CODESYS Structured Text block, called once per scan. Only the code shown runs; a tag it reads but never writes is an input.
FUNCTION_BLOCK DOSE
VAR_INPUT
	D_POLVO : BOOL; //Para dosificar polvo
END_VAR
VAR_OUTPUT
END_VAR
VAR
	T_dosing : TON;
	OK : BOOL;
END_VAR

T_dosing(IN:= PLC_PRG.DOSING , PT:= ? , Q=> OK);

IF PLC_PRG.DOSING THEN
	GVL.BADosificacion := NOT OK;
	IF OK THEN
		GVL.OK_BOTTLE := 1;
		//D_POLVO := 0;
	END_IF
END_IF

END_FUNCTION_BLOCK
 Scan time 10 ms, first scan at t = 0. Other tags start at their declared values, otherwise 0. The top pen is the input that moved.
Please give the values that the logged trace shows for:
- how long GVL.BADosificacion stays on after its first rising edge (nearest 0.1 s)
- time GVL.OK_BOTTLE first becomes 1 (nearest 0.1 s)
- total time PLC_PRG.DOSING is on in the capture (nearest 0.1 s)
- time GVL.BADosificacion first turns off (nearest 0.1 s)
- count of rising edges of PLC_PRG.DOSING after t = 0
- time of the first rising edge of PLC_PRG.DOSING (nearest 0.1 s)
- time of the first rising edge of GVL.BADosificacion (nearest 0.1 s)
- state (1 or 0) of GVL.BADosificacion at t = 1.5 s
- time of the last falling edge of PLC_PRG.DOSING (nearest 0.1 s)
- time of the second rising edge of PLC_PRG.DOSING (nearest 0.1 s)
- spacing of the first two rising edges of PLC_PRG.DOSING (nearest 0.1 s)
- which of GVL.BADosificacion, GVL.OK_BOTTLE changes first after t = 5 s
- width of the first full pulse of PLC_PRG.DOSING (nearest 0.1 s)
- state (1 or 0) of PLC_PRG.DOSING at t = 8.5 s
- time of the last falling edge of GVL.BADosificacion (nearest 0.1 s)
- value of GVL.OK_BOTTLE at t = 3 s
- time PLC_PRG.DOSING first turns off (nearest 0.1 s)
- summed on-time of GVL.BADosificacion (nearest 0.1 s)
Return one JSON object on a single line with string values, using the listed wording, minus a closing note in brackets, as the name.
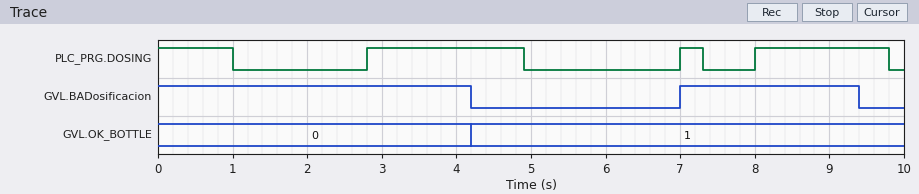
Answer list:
{"how long GVL.BADosificacion stays on after its first rising edge": "2.4 s", "time GVL.OK_BOTTLE first becomes 1": "4.2 s", "total time PLC_PRG.DOSING is on in the capture": "5.2 s", "time GVL.BADosificacion first turns off": "4.2 s", "count of rising edges of PLC_PRG.DOSING after t = 0": "3", "time of the first rising edge of PLC_PRG.DOSING": "2.8 s", "time of the first rising edge of GVL.BADosificacion": "7.0 s", "state (1 or 0) of GVL.BADosificacion at t = 1.5 s": "1", "time of the last falling edge of PLC_PRG.DOSING": "9.8 s", "time of the second rising edge of PLC_PRG.DOSING": "7.0 s", "spacing of the first two rising edges of PLC_PRG.DOSING": "4.2 s", "which of GVL.BADosificacion, GVL.OK_BOTTLE changes first after t = 5 s": "GVL.BADosificacion", "width of the first full pulse of PLC_PRG.DOSING": "2.1 s", "state (1 or 0) of PLC_PRG.DOSING at t = 8.5 s": "1", "time of the last falling edge of GVL.BADosificacion": "9.4 s", "value of GVL.OK_BOTTLE at t = 3 s": "0", "time PLC_PRG.DOSING first turns off": "1.0 s", "summed on-time of GVL.BADosificacion": "6.6 s"}
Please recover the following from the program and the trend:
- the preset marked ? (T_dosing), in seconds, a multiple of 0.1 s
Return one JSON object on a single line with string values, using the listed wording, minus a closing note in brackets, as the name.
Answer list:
{"the preset marked ? (T_dosing), in seconds, a multiple of 0.1 s": "1.4 s"}
